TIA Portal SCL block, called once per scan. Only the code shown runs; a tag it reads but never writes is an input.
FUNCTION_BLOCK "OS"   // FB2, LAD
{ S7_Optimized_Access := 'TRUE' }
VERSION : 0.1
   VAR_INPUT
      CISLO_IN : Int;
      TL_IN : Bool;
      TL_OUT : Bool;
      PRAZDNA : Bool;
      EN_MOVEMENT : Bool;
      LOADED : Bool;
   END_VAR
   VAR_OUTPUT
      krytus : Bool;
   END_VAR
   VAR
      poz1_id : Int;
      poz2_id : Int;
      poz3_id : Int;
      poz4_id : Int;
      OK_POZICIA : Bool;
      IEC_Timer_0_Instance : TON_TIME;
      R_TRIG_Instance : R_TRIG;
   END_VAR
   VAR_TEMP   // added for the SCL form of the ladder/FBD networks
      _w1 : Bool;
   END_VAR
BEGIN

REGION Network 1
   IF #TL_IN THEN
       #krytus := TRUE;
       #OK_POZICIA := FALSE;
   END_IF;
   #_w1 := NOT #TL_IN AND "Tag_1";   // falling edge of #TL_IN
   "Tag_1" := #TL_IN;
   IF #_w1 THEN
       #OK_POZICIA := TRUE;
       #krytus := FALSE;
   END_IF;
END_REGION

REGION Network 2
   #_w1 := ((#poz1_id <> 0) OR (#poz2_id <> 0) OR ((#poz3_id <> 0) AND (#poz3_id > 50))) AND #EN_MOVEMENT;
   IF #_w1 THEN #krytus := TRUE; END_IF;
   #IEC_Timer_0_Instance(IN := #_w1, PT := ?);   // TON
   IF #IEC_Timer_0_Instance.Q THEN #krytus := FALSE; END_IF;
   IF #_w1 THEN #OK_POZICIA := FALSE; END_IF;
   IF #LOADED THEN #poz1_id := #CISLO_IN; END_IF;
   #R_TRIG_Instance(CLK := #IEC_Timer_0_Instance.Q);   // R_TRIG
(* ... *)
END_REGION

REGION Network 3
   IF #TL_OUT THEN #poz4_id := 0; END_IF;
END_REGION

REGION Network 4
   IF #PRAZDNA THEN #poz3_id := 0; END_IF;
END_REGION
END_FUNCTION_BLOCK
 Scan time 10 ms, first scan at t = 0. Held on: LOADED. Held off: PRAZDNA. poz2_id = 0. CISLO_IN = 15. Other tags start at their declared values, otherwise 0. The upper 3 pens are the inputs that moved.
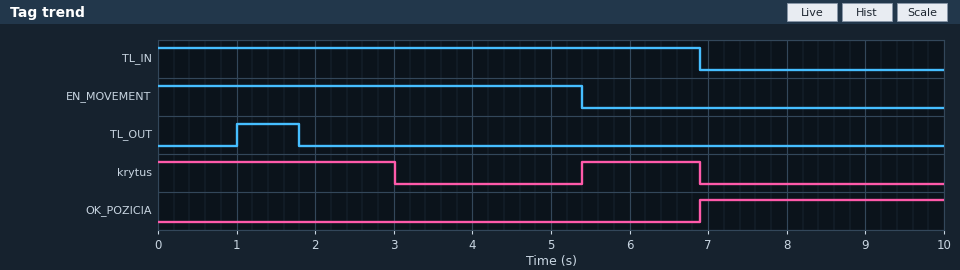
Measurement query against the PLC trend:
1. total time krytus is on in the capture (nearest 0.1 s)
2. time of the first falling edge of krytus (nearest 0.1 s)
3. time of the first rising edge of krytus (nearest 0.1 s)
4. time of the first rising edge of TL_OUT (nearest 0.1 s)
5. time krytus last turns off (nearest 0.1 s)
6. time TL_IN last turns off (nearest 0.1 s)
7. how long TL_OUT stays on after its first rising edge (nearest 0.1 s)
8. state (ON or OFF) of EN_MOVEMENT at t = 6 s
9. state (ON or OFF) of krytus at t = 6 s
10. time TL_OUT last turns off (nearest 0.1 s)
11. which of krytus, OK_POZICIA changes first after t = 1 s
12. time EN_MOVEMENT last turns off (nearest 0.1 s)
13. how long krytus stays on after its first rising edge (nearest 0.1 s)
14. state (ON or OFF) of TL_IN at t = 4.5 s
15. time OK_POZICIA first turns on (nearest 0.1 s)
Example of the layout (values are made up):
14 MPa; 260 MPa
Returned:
4.5 s; 3.0 s; 5.4 s; 1.0 s; 6.9 s; 6.9 s; 0.8 s; OFF; ON; 1.8 s; krytus; 5.4 s; 1.5 s; ON; 6.9 s
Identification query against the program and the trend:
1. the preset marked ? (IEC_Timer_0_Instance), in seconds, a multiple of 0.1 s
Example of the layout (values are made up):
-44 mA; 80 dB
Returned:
3.0 s
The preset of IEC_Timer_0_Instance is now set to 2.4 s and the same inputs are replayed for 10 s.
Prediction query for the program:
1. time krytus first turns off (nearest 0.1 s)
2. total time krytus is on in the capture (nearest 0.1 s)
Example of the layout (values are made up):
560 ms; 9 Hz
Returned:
2.4 s; 3.9 s
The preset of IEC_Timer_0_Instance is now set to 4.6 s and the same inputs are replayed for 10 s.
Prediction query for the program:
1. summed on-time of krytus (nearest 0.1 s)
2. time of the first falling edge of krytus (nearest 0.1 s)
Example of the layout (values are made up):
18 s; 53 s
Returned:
6.1 s; 4.6 s
